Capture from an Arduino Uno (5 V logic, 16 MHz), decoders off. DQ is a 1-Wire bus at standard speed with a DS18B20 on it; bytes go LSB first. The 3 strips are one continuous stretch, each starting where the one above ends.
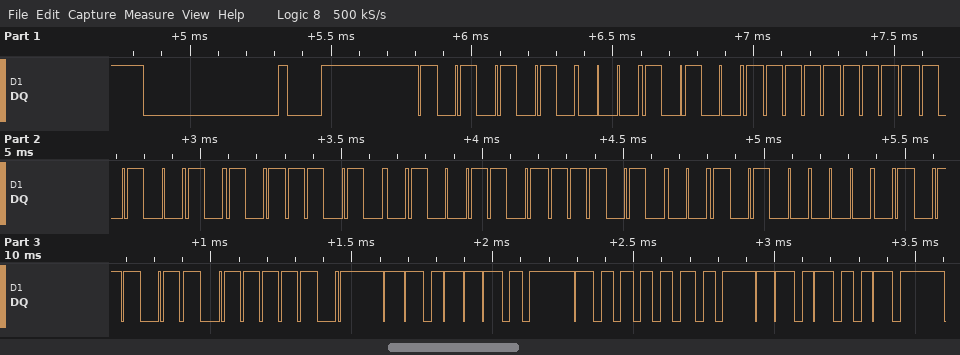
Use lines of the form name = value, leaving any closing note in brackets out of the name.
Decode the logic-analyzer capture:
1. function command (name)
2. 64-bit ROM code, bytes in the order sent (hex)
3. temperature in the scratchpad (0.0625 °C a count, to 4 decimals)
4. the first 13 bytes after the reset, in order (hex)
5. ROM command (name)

function command = Read Scratchpad
64-bit ROM code, bytes in the order sent = 28 FF 4B 5D B2 17 05 DA
temperature in the scratchpad = 19.6875 °C
the first 13 bytes after the reset, in order = 55 28 FF 4B 5D B2 17 05 DA BE 3B 01 4B
ROM command = Match ROM
